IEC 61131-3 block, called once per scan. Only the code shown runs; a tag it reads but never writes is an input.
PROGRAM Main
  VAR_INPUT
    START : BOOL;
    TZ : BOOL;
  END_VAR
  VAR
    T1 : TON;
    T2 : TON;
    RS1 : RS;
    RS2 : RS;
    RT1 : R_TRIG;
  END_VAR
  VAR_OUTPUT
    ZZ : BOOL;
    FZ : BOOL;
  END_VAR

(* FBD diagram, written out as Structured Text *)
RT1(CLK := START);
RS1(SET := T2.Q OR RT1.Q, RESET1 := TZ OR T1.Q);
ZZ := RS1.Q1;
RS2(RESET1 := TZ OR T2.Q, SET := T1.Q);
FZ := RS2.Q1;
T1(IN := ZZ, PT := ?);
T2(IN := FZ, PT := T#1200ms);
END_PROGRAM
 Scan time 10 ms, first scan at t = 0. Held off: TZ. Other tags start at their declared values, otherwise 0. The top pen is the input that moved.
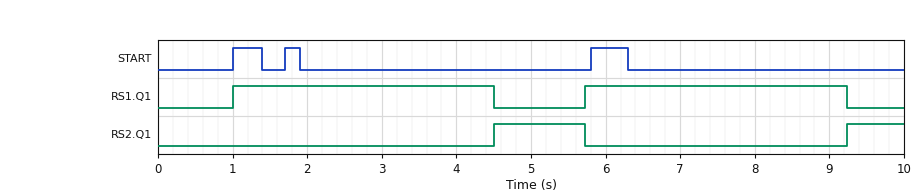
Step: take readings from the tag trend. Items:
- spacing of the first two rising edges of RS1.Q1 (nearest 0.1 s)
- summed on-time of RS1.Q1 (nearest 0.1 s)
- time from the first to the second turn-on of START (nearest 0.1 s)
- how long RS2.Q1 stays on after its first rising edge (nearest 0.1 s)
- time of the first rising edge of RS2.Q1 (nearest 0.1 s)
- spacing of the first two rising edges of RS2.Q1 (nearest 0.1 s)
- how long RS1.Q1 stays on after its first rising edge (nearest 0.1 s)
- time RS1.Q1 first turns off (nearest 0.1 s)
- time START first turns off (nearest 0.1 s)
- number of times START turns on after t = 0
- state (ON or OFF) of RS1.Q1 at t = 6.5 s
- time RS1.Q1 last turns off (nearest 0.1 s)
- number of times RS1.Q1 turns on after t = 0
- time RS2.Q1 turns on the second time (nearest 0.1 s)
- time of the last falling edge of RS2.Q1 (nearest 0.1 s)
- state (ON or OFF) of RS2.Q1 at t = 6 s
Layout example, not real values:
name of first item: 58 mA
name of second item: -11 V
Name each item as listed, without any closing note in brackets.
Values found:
spacing of the first two rising edges of RS1.Q1: 4.7 s
summed on-time of RS1.Q1: 7.0 s
time from the first to the second turn-on of START: 0.7 s
how long RS2.Q1 stays on after its first rising edge: 1.2 s
time of the first rising edge of RS2.Q1: 4.5 s
spacing of the first two rising edges of RS2.Q1: 4.7 s
how long RS1.Q1 stays on after its first rising edge: 3.5 s
time RS1.Q1 first turns off: 4.5 s
time START first turns off: 1.4 s
number of times START turns on after t = 0: 3
state (ON or OFF) of RS1.Q1 at t = 6.5 s: ON
time RS1.Q1 last turns off: 9.2 s
number of times RS1.Q1 turns on after t = 0: 2
time RS2.Q1 turns on the second time: 9.2 s
time of the last falling edge of RS2.Q1: 5.7 s
state (ON or OFF) of RS2.Q1 at t = 6 s: OFF
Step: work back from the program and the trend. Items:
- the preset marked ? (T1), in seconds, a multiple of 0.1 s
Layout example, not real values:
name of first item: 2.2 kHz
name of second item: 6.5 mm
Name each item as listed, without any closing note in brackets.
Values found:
the preset marked ? (T1), in seconds, a multiple of 0.1 s: 3.5 s
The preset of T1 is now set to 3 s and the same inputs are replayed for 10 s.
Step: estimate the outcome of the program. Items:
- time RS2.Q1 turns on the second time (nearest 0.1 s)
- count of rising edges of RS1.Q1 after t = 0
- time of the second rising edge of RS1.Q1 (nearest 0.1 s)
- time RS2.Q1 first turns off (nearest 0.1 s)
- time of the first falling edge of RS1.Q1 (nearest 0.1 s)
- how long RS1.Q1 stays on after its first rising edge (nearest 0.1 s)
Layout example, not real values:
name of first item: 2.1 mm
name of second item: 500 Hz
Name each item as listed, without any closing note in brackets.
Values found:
time RS2.Q1 turns on the second time: 8.2 s
count of rising edges of RS1.Q1 after t = 0: 3
time of the second rising edge of RS1.Q1: 5.2 s
time RS2.Q1 first turns off: 5.2 s
time of the first falling edge of RS1.Q1: 4.0 s
how long RS1.Q1 stays on after its first rising edge: 3.0 s
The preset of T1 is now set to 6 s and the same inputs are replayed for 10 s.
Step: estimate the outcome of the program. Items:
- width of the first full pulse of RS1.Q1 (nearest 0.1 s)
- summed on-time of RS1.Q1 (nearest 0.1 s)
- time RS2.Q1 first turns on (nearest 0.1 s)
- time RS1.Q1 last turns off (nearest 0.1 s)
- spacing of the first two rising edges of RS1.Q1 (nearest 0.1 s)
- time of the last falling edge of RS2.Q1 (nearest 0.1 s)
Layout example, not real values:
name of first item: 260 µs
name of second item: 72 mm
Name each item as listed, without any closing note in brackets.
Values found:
width of the first full pulse of RS1.Q1: 6.0 s
summed on-time of RS1.Q1: 7.8 s
time RS2.Q1 first turns on: 7.0 s
time RS1.Q1 last turns off: 7.0 s
spacing of the first two rising edges of RS1.Q1: 7.2 s
time of the last falling edge of RS2.Q1: 8.2 s
